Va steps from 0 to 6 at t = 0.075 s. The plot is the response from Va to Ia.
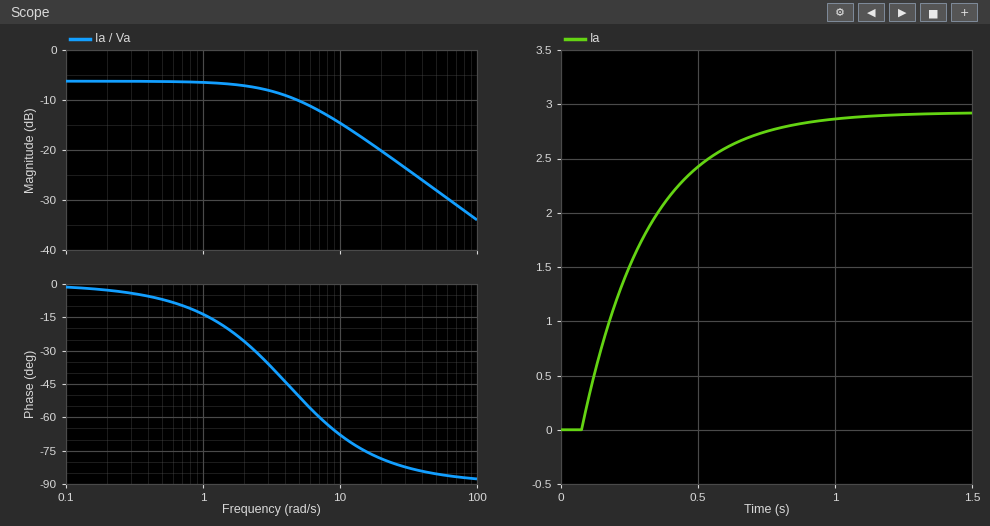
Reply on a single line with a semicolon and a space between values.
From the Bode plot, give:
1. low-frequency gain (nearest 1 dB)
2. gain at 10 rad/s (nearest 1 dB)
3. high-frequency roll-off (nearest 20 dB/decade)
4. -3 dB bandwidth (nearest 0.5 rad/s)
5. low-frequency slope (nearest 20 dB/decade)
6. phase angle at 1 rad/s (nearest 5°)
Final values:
-6 dB; -15 dB; -20 dB/decade; 4.0 rad/s; 0 dB/decade; -15°
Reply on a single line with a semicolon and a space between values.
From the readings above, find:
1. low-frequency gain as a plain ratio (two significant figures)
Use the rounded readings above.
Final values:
0.50
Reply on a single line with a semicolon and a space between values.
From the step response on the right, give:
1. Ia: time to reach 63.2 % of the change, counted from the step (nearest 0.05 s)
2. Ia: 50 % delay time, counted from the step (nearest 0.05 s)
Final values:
0.25 s; 0.15 s
